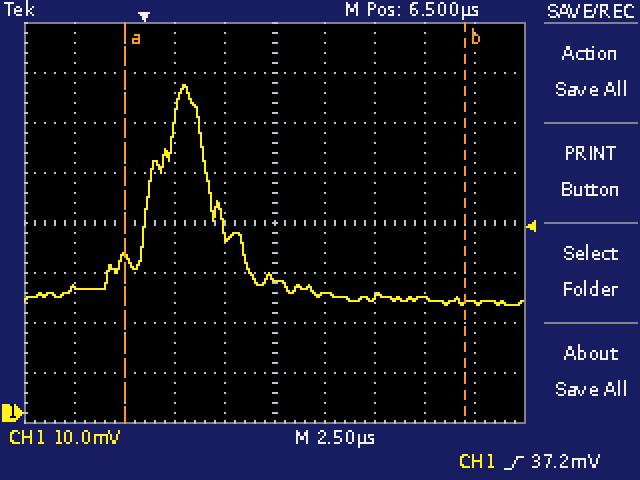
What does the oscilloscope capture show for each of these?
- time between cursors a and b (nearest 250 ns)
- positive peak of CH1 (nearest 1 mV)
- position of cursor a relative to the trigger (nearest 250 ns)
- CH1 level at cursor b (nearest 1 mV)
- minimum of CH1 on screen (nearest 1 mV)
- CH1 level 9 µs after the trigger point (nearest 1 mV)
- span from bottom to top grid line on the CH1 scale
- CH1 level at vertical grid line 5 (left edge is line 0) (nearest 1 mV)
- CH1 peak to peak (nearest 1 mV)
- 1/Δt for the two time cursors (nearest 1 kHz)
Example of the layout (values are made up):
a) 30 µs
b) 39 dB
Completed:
a) 17.00 µs
b) 66 mV
c) -1.00 µs
d) 22 mV
e) 22 mV
f) 24 mV
g) 80 mV
h) 27 mV
i) 44 mV
j) 59 kHz
